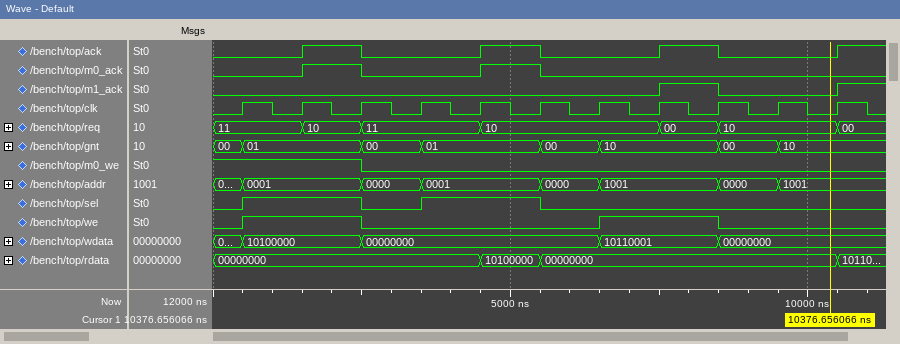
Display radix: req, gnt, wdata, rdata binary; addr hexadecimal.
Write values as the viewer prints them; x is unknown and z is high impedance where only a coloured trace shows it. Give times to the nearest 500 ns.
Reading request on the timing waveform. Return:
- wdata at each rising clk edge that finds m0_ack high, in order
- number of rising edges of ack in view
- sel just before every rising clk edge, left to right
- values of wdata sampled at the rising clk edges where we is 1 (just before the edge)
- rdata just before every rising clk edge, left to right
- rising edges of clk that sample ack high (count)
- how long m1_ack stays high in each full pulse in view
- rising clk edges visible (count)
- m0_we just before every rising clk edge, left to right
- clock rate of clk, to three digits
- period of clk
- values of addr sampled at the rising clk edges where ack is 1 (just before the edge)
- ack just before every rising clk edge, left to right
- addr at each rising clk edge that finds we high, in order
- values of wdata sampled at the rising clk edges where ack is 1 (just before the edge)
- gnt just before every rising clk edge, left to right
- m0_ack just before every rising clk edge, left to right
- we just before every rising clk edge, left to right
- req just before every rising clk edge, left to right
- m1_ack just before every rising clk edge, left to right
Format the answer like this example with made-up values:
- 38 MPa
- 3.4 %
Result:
- 10100000, 00000000
- 4
- 0 1 1 0 1 1 0 0 0 0 0
- 10100000, 10100000, 10110001, 10110001
- 00000000, 00000000, 00000000, 00000000, 00000000, 10100000, 00000000, 00000000, 00000000, 00000000, 00000000
- 3
- 1000 ns
- 11
- 1 1 1 0 0 0 0 0 0 0 0
- 1.00 MHz
- 1000 ns
- 0001, 0001, 1001
- 0 0 1 0 0 1 0 0 1 0 0
- 0001, 0001, 1001, 1001
- 10100000, 00000000, 10110001
- 00, 01, 01, 00, 01, 01, 00, 10, 10, 00, 10
- 0 0 1 0 0 1 0 0 0 0 0
- 0 1 1 0 0 0 0 1 1 0 0
- 11, 11, 10, 11, 11, 10, 10, 10, 00, 10, 10
- 0 0 0 0 0 0 0 0 1 0 0
